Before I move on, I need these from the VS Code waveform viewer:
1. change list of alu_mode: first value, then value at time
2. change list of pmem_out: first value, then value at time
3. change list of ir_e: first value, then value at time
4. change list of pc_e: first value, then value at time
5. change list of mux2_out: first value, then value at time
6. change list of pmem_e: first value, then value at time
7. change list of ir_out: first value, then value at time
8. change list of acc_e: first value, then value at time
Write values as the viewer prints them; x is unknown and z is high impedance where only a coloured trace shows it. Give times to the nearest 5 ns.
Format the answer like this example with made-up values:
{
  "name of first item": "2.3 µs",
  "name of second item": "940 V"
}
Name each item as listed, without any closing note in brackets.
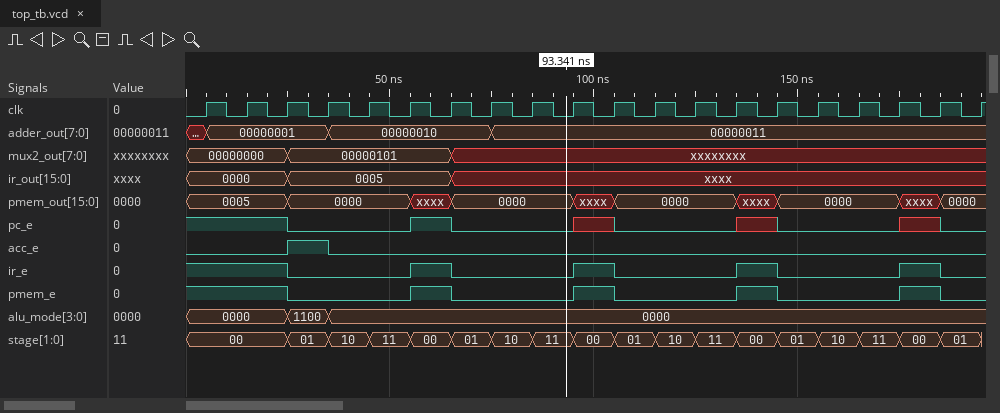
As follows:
{
  "change list of alu_mode: first value, then value at time": "0000, 1100 at 25 ns, 0000 at 35 ns",
  "change list of pmem_out: first value, then value at time": "0005, 0000 at 25 ns, xxxx at 55 ns, 0000 at 65 ns, xxxx at 95 ns, 0000 at 105 ns, xxxx at 135 ns, 0000 at 145 ns, xxxx at 175 ns, 0000 at 185 ns",
  "change list of ir_e: first value, then value at time": "1, 0 at 25 ns, 1 at 55 ns, 0 at 65 ns, 1 at 95 ns, 0 at 105 ns, 1 at 135 ns, 0 at 145 ns, 1 at 175 ns, 0 at 185 ns",
  "change list of pc_e: first value, then value at time": "1, 0 at 25 ns, 1 at 55 ns, 0 at 65 ns, x at 95 ns, 0 at 105 ns, x at 135 ns, 0 at 145 ns, x at 175 ns, 0 at 185 ns",
  "change list of mux2_out: first value, then value at time": "00000000, 00000101 at 25 ns, xxxxxxxx at 65 ns",
  "change list of pmem_e: first value, then value at time": "1, 0 at 25 ns, 1 at 55 ns, 0 at 65 ns, 1 at 95 ns, 0 at 105 ns, 1 at 135 ns, 0 at 145 ns, 1 at 175 ns, 0 at 185 ns",
  "change list of ir_out: first value, then value at time": "0000, 0005 at 25 ns, xxxx at 65 ns",
  "change list of acc_e: first value, then value at time": "0, 1 at 25 ns, 0 at 35 ns"
}
